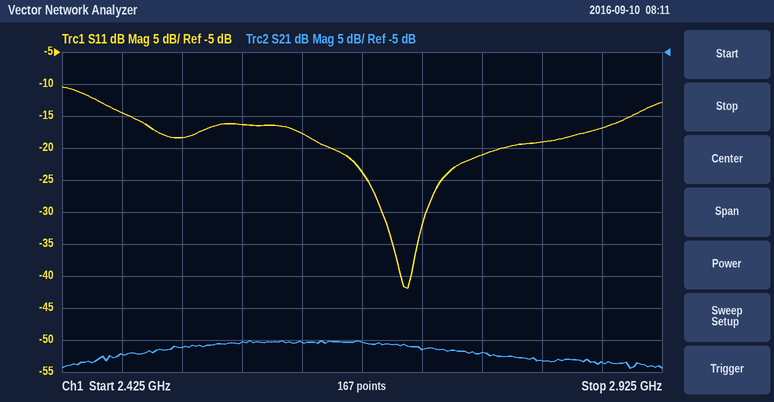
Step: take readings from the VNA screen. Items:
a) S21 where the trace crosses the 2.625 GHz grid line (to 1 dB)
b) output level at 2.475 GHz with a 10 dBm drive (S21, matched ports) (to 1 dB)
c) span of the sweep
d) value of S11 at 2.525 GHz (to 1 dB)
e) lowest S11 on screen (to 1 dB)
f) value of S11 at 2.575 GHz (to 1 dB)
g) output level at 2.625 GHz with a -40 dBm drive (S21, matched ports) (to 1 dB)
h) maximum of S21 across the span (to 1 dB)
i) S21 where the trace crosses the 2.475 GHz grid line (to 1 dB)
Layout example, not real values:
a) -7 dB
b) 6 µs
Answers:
a) -50 dB
b) -42 dBm
c) 500 MHz
d) -18 dB
e) -42 dB
f) -16 dB
g) -90 dBm
h) -50 dB
i) -52 dB
